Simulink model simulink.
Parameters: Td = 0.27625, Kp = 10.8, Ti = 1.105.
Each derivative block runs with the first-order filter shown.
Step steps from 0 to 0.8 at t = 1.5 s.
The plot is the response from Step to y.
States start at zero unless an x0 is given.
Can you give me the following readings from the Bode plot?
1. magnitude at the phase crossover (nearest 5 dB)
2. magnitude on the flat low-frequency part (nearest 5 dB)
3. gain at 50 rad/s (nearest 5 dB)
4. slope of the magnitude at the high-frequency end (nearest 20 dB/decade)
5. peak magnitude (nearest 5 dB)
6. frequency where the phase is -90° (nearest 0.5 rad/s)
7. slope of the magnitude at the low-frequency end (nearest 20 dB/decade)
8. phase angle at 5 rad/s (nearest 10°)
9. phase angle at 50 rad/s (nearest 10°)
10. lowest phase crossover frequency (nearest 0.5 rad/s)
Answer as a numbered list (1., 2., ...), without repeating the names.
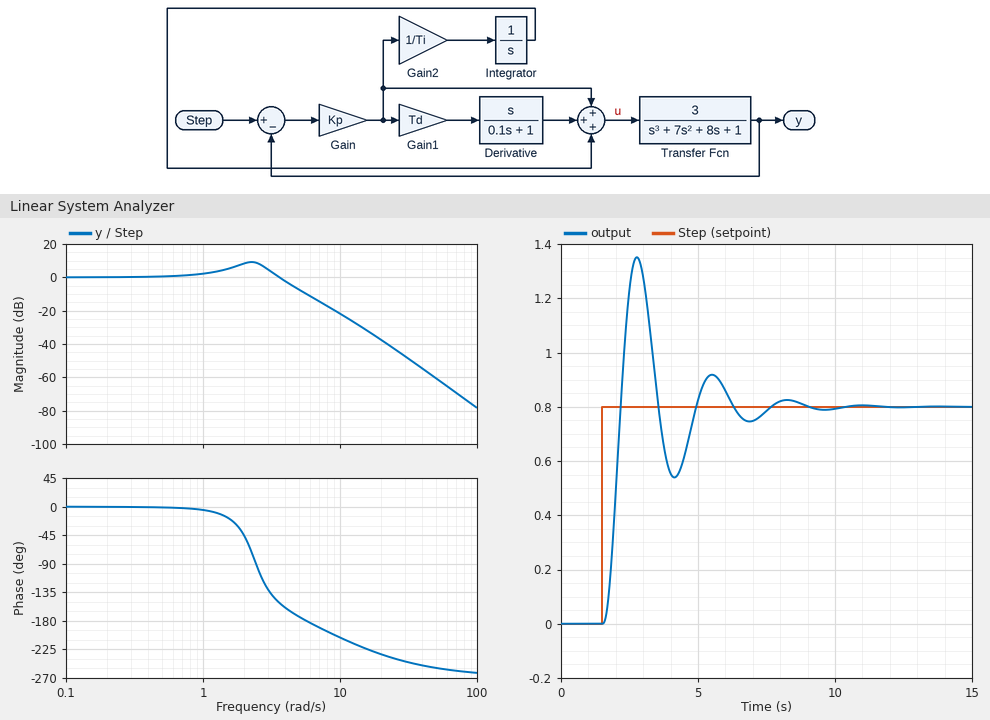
1. -10 dB
2. 0 dB
3. -60 dB
4. -60 dB/decade
5. 10 dB
6. 2.5 rad/s
7. 0 dB/decade
8. -170°
9. -250°
10. 5.5 rad/s
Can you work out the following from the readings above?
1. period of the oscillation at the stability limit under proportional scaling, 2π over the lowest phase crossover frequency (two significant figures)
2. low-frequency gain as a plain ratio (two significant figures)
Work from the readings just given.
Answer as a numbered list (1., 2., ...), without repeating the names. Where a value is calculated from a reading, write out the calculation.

1. 2π / 5.5 = 1.1 s
2. 10^(0 / 20) = 1.0
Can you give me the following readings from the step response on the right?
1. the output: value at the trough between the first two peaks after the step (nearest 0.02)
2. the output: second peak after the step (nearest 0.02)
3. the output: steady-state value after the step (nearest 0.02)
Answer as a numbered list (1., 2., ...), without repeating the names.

1. 0.54
2. 0.92
3. 0.80
